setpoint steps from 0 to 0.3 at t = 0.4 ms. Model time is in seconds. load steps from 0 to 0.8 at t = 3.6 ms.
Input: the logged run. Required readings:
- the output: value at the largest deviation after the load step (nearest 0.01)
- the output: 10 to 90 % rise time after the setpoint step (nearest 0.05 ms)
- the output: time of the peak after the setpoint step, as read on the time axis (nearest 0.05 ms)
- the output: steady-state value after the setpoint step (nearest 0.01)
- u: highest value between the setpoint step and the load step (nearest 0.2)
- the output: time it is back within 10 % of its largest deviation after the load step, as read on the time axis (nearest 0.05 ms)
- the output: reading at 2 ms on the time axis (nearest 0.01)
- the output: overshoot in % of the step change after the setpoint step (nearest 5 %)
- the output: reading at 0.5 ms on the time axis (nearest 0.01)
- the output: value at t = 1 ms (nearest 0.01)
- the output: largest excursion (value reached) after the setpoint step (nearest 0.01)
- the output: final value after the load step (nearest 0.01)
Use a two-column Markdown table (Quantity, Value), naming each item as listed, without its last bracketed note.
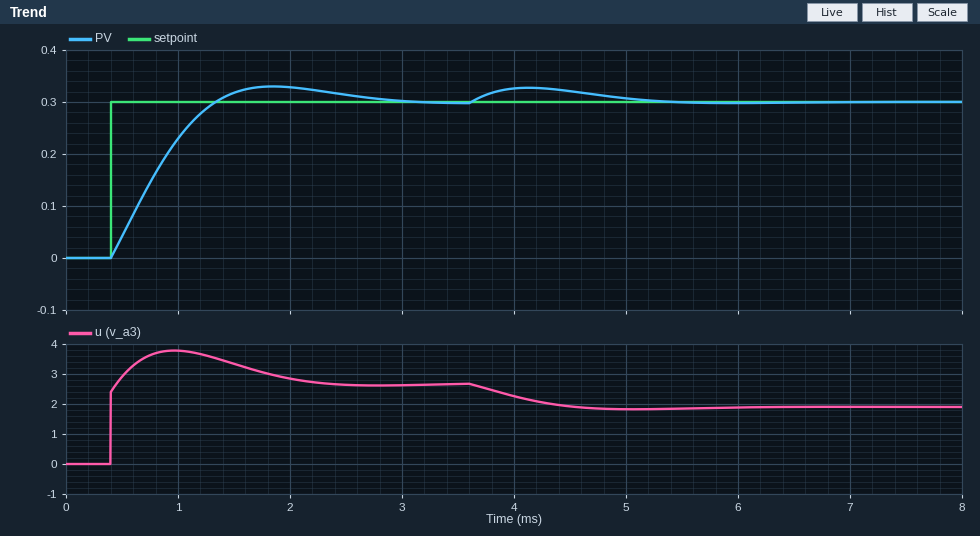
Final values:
| Quantity | Value |
|---|---|
| the output: value at the largest deviation after the load step | 0.33 |
| the output: 10 to 90 % rise time after the setpoint step | 0.70 ms |
| the output: time of the peak after the setpoint step, as read on the time axis | 1.85 ms |
| the output: steady-state value after the setpoint step | 0.30 |
| u: highest value between the setpoint step and the load step | 3.8 |
| the output: time it is back within 10 % of its largest deviation after the load step, as read on the time axis | 5.20 ms |
| the output: reading at 2 ms on the time axis | 0.33 |
| the output: overshoot in % of the step change after the setpoint step | 10 % |
| the output: reading at 0.5 ms on the time axis | 0.04 |
| the output: value at t = 1 ms | 0.23 |
| the output: largest excursion (value reached) after the setpoint step | 0.33 |
| the output: final value after the load step | 0.30 |
